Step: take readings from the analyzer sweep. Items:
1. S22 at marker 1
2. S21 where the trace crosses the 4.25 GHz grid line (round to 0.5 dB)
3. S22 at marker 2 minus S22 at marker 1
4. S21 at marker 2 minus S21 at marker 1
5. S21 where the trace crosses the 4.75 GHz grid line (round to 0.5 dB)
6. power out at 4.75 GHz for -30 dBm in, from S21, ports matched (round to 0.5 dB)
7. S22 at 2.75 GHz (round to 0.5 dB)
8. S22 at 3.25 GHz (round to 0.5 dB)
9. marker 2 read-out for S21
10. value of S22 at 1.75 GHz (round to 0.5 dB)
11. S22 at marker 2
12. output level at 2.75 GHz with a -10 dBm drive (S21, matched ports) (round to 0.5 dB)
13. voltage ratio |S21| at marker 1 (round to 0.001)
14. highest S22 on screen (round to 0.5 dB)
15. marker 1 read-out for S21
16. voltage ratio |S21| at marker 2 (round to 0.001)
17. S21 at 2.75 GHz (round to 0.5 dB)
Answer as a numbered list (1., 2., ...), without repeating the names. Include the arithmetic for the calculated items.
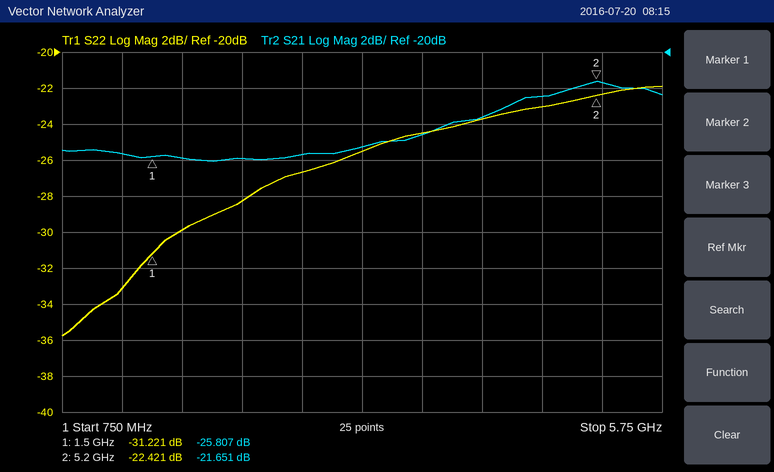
1. -31.221 dB
2. -23.5 dB
3. -22.421 − (-31.221) = 8.800 dB
4. -21.651 − (-25.807) = 4.156 dB
5. -22.5 dB
6. -30 dBm + (-22.5 dB) = -52.5 dBm
7. -26.5 dB
8. -25.5 dB
9. -21.651 dB
10. -30.0 dB
11. -22.421 dB
12. -10 dBm + (-25.5 dB) = -35.5 dBm
13. 10^(-25.807/20) ≈ 0.051
14. -22.0 dB
15. -25.807 dB
16. 10^(-21.651/20) ≈ 0.083
17. -25.5 dB
